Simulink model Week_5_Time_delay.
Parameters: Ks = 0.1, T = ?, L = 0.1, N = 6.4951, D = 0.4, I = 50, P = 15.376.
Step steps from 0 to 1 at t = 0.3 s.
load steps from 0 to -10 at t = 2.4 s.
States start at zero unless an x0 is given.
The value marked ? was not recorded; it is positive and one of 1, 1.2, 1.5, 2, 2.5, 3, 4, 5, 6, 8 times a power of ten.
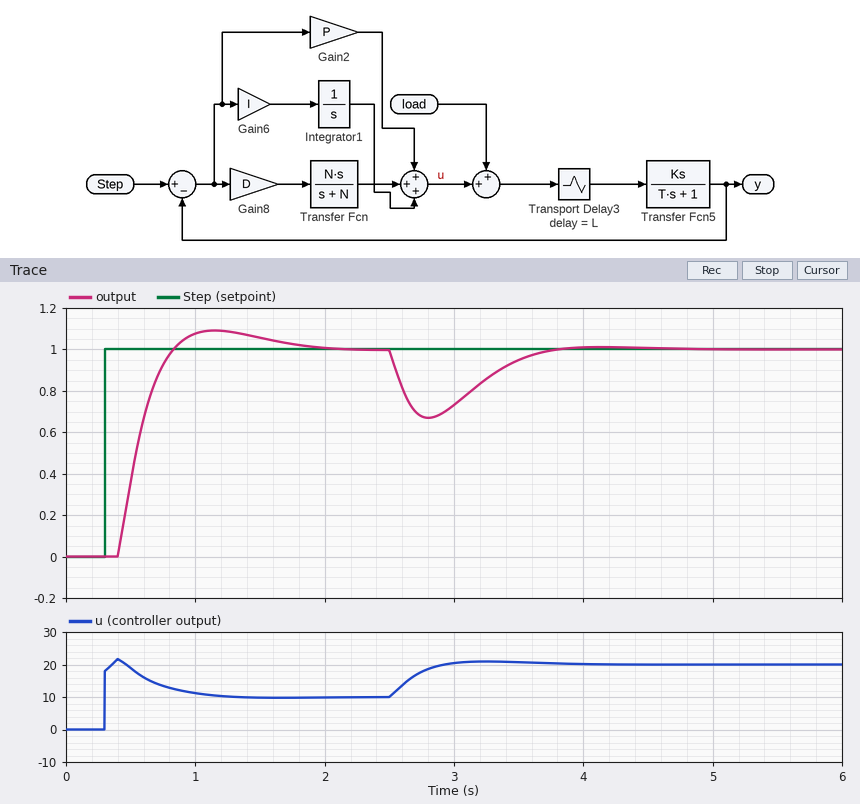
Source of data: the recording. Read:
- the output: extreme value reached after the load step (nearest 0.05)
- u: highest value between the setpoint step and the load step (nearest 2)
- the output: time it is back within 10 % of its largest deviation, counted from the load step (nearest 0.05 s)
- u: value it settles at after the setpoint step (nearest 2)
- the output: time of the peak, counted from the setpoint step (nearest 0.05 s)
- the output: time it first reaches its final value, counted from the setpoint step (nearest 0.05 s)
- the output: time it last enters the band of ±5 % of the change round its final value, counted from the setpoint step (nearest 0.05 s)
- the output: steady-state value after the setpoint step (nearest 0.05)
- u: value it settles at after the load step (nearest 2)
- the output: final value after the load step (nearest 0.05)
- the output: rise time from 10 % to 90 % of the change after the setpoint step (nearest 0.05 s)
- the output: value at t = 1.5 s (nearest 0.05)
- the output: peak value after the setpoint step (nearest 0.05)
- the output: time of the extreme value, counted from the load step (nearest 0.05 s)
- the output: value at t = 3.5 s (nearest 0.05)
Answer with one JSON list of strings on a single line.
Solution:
["0.65", "22", "1.20 s", "10", "0.85 s", "0.55 s", "1.25 s", "1.00", "20", "1.00", "0.30 s", "1.05", "1.10", "0.40 s", "0.95"]
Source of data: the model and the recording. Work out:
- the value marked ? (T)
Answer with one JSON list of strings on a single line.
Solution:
["0.5"]
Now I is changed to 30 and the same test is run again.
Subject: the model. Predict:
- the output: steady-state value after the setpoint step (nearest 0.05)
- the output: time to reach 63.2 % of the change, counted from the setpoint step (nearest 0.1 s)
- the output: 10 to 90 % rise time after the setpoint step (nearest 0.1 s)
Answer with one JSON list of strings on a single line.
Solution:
["1.00", "0.3 s", "0.5 s"]
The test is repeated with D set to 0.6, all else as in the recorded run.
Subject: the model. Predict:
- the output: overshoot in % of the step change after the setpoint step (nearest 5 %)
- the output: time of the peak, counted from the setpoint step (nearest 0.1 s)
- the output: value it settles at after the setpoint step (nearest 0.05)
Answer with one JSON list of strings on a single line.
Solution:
["10 %", "0.9 s", "1.00"]
